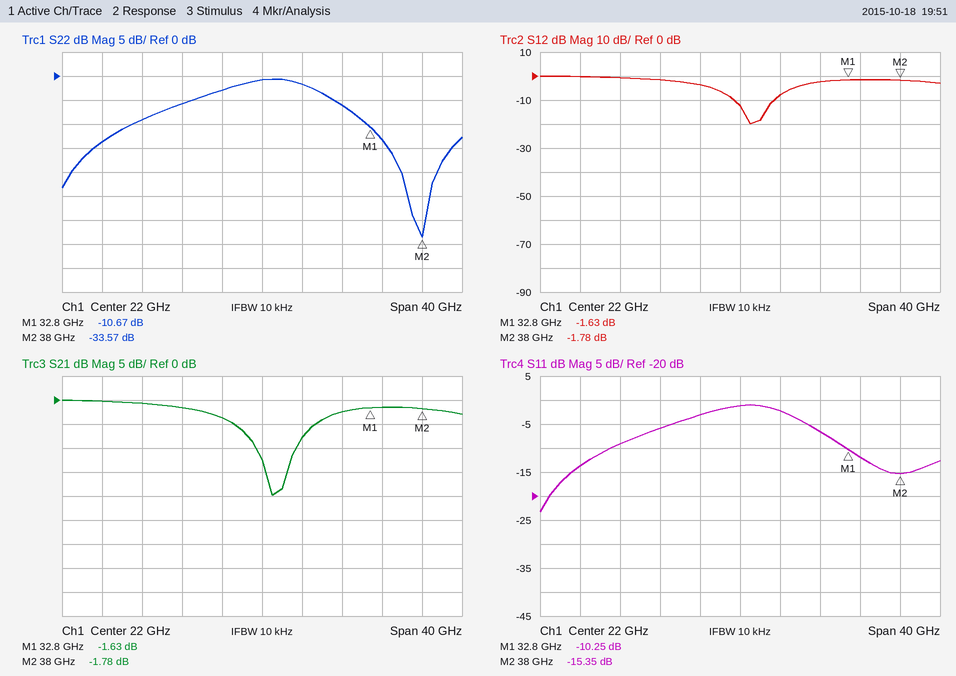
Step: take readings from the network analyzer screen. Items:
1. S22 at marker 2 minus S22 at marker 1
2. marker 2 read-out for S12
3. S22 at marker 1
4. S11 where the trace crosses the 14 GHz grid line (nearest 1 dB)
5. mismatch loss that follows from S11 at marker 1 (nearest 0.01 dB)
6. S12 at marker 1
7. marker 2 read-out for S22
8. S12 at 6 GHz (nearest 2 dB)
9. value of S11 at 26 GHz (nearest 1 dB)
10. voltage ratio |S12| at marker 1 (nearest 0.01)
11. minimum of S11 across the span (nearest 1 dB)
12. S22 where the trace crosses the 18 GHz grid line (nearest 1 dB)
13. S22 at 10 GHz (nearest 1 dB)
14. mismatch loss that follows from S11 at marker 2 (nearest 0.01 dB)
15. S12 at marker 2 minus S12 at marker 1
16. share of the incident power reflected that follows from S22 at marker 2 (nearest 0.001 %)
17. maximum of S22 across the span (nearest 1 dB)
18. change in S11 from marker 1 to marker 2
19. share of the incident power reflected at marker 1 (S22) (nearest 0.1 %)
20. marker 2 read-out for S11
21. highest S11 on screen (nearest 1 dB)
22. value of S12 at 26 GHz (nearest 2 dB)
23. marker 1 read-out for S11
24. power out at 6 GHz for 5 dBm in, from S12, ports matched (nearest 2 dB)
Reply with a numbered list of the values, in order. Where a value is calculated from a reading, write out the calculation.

1. -33.57 − (-10.67) = -22.90 dB
2. -1.78 dB
3. -10.67 dB
4. -6 dB
5. −10 log10(1 − 10^(-10.25/10)) ≈ 0.43 dB
6. -1.63 dB
7. -33.57 dB
8. 0 dB
9. -2 dB
10. 10^(-1.63/20) ≈ 0.83
11. -23 dB
12. -3 dB
13. -9 dB
14. −10 log10(1 − 10^(-15.35/10)) ≈ 0.13 dB
15. -1.78 − (-1.63) = -0.15 dB
16. 10^(-33.57/10) ≈ 0.044 %
17. -1 dB
18. -15.35 − (-10.25) = -5.10 dB
19. 10^(-10.67/10) ≈ 8.6 %
20. -15.35 dB
21. -1 dB
22. -8 dB
23. -10.25 dB
24. 5 dBm + (0 dB) = 4 dBm
